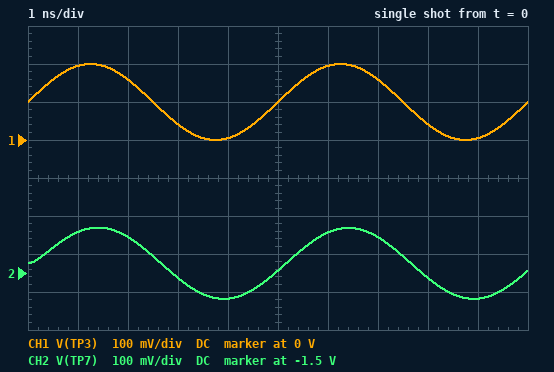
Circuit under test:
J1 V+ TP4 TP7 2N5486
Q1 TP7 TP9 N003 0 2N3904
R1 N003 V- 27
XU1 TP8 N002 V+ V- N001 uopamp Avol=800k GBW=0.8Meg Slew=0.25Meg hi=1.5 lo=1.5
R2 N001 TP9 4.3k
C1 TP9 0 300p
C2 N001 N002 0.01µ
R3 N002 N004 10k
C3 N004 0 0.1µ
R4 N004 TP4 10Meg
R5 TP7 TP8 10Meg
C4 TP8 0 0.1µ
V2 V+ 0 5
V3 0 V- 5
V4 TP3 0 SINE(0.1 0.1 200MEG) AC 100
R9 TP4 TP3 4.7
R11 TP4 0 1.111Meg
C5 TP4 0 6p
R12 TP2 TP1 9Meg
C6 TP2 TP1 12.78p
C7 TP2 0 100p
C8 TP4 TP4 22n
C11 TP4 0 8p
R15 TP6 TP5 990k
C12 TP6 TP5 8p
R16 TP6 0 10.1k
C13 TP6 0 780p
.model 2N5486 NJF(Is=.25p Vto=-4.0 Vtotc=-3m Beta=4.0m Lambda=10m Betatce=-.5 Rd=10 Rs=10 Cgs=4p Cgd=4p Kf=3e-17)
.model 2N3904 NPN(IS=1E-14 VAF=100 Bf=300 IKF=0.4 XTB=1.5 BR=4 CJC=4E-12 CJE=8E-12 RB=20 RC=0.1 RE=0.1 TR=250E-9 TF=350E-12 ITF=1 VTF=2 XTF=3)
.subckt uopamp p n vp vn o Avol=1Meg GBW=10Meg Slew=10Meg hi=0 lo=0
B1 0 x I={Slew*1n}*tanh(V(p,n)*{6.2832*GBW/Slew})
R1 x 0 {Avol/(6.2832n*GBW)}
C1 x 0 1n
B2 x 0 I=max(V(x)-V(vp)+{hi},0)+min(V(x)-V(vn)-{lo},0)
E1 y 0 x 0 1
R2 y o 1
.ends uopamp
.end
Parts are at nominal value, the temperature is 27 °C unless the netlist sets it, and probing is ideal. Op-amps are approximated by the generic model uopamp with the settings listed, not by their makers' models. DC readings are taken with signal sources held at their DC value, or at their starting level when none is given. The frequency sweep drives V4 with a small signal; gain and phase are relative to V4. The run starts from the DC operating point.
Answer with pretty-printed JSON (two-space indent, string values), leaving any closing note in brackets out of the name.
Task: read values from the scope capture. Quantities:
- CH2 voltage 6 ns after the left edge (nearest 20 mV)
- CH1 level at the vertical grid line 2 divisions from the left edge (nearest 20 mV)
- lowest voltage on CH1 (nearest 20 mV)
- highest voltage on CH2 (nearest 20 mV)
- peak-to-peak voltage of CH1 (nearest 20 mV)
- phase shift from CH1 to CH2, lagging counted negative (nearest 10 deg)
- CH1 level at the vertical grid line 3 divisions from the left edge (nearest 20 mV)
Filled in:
{
  "CH2 voltage 6 ns after the left edge": "-1.40 V",
  "CH1 level at the vertical grid line 2 divisions from the left edge": "160 mV",
  "lowest voltage on CH1": "0 V",
  "highest voltage on CH2": "-1.38 V",
  "peak-to-peak voltage of CH1": "200 mV",
  "phase shift from CH1 to CH2, lagging counted negative": "-10 deg",
  "CH1 level at the vertical grid line 3 divisions from the left edge": "40 mV"
}
